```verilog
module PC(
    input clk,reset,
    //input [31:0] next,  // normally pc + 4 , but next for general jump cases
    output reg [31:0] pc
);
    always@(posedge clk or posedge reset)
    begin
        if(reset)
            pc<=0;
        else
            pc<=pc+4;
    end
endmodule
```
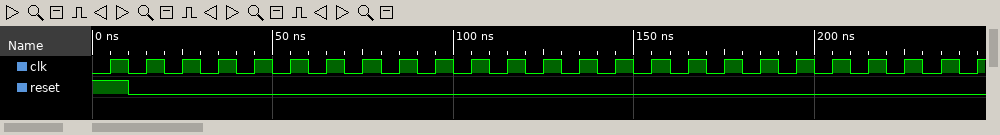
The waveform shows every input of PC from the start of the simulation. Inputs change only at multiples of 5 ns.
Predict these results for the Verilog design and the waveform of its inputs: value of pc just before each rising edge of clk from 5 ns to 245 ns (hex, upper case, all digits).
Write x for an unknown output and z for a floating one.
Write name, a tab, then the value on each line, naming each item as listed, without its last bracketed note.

value of pc just before each rising edge of clk from 5 ns to 245 ns	00000000, 00000000, 00000004, 00000008, 0000000C, 00000010, 00000014, 00000018, 0000001C, 00000020, 00000024, 00000028, 0000002C, 00000030, 00000034, 00000038, 0000003C, 00000040, 00000044, 00000048, 0000004C, 00000050, 00000054, 00000058, 0000005C
